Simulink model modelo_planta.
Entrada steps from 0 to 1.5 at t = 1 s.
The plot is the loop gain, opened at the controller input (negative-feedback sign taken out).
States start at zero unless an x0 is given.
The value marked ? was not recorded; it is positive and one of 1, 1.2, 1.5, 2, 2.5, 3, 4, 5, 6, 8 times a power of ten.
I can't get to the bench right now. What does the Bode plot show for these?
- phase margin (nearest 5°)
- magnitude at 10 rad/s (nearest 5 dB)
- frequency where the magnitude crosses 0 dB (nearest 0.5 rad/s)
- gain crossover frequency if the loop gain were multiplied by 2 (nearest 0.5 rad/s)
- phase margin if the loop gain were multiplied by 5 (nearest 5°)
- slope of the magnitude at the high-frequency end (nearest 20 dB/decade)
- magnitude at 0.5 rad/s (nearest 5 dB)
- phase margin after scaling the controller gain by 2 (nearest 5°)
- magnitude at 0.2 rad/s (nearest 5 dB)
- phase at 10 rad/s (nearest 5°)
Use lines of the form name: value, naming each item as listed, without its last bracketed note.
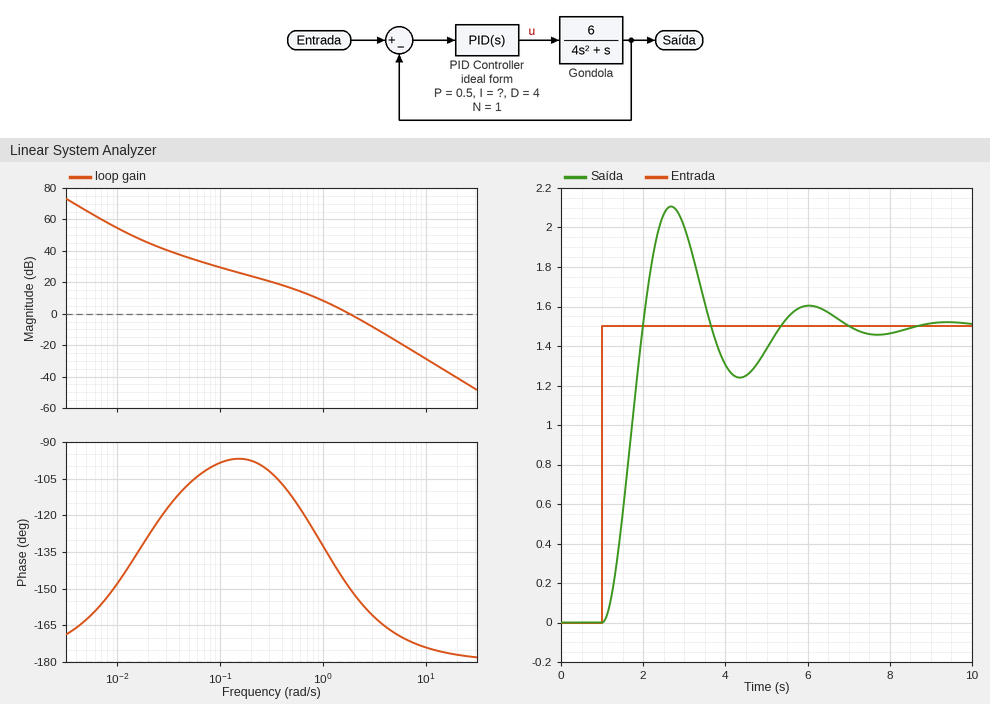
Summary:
phase margin: 30°
magnitude at 10 rad/s: -30 dB
frequency where the magnitude crosses 0 dB: 2.0 rad/s
gain crossover frequency if the loop gain were multiplied by 2: 2.5 rad/s
phase margin if the loop gain were multiplied by 5: 15°
slope of the magnitude at the high-frequency end: -40 dB/decade
magnitude at 0.5 rad/s: 15 dB
phase margin after scaling the controller gain by 2: 20°
magnitude at 0.2 rad/s: 25 dB
phase at 10 rad/s: -175°
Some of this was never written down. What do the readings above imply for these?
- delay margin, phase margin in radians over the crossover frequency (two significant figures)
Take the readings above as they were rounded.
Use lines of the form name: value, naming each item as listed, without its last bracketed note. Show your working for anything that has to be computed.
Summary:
delay margin, phase margin in radians over the crossover frequency: 30 × π / 180 / 2 = 0.26 s
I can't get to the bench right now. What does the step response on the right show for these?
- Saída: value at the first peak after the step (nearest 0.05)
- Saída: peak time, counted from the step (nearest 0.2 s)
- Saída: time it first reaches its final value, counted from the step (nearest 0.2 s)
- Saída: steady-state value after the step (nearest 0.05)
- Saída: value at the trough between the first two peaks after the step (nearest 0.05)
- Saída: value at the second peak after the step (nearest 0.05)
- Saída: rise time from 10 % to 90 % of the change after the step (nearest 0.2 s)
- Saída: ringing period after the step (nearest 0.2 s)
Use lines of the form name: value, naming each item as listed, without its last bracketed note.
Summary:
Saída: value at the first peak after the step: 2.10
Saída: peak time, counted from the step: 1.6 s
Saída: time it first reaches its final value, counted from the step: 1.0 s
Saída: steady-state value after the step: 1.50
Saída: value at the trough between the first two peaks after the step: 1.25
Saída: value at the second peak after the step: 1.60
Saída: rise time from 10 % to 90 % of the change after the step: 0.6 s
Saída: ringing period after the step: 3.4 s
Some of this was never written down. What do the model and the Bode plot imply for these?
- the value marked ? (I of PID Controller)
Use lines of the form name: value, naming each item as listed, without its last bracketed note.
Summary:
the value marked ?: 0.015
